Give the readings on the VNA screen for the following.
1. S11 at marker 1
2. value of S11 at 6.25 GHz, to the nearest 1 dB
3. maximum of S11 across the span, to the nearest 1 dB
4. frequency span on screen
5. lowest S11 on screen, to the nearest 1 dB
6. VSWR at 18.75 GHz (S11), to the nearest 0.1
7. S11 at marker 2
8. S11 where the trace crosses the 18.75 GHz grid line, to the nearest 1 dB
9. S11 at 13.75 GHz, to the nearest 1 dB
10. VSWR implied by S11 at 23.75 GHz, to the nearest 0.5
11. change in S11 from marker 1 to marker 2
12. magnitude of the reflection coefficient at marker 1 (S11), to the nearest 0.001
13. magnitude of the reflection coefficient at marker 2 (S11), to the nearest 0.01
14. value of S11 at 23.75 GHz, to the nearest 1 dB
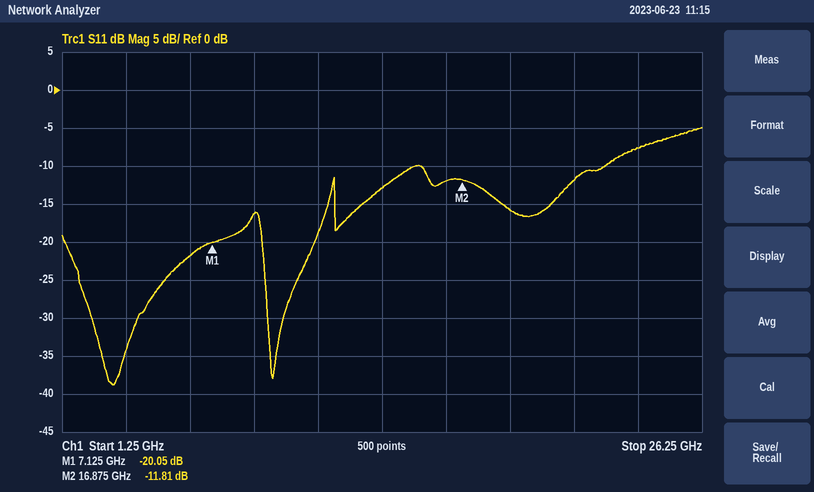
-20.05 dB
-22 dB
-5 dB
25 GHz
-39 dB
1.4
-11.81 dB
-16 dB
-13 dB
2.5
8.24 dB
0.099
0.26
-8 dB
